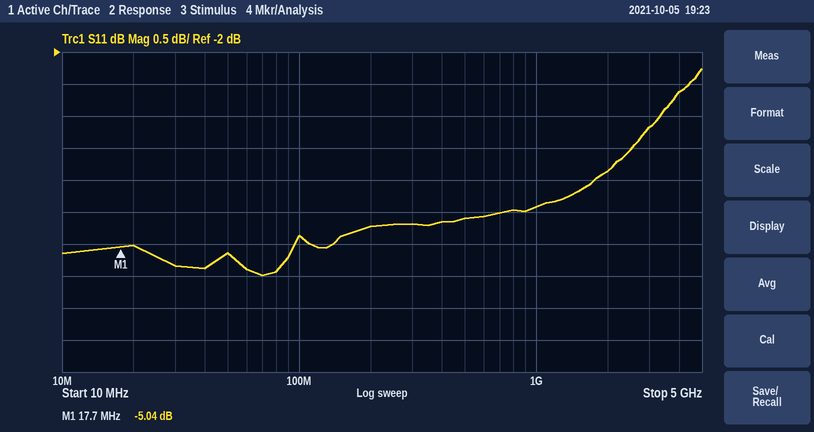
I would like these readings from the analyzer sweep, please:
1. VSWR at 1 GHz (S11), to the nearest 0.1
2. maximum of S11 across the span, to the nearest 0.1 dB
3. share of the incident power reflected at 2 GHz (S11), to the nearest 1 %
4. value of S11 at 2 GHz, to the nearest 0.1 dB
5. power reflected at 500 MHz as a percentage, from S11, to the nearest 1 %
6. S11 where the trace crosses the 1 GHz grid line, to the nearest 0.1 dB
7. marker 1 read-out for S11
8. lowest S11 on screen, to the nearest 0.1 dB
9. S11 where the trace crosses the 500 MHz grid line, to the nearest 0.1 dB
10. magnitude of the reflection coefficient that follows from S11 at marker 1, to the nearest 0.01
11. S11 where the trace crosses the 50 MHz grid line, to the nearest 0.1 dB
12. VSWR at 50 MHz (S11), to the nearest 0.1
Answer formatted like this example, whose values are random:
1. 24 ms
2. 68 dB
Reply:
1. 4.0
2. -2.3 dB
3. 41 %
4. -3.9 dB
5. 35 %
6. -4.4 dB
7. -5.04 dB
8. -5.5 dB
9. -4.6 dB
10. 0.56
11. -5.1 dB
12. 3.5
